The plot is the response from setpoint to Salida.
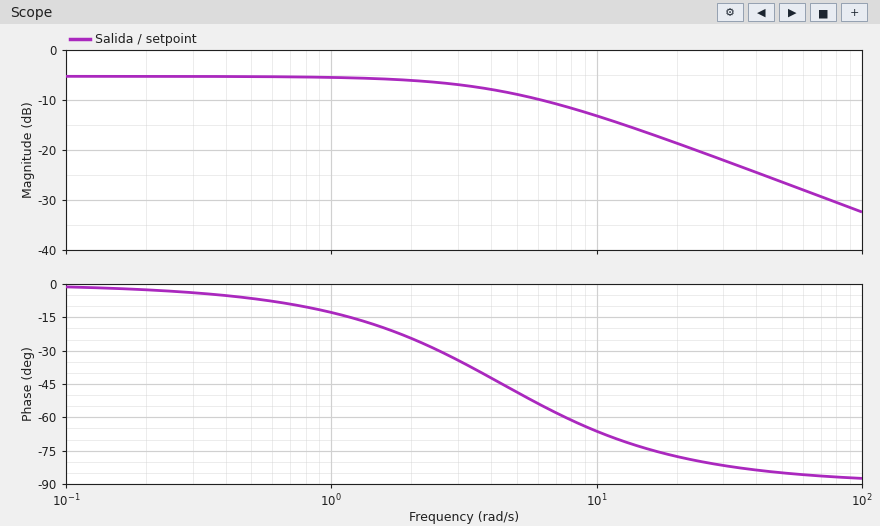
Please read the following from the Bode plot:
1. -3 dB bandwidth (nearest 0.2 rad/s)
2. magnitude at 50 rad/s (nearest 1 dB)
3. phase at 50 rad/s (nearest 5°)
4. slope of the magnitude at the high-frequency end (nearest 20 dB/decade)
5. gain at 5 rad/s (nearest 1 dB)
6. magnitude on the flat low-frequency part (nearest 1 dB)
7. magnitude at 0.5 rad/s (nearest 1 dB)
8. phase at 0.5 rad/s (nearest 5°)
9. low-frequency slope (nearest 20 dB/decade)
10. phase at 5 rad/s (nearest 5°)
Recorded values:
4.4 rad/s
-26 dB
-85°
-20 dB/decade
-9 dB
-5 dB
-5 dB
-5°
0 dB/decade
-50°
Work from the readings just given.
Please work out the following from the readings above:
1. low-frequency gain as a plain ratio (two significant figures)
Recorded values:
0.56
